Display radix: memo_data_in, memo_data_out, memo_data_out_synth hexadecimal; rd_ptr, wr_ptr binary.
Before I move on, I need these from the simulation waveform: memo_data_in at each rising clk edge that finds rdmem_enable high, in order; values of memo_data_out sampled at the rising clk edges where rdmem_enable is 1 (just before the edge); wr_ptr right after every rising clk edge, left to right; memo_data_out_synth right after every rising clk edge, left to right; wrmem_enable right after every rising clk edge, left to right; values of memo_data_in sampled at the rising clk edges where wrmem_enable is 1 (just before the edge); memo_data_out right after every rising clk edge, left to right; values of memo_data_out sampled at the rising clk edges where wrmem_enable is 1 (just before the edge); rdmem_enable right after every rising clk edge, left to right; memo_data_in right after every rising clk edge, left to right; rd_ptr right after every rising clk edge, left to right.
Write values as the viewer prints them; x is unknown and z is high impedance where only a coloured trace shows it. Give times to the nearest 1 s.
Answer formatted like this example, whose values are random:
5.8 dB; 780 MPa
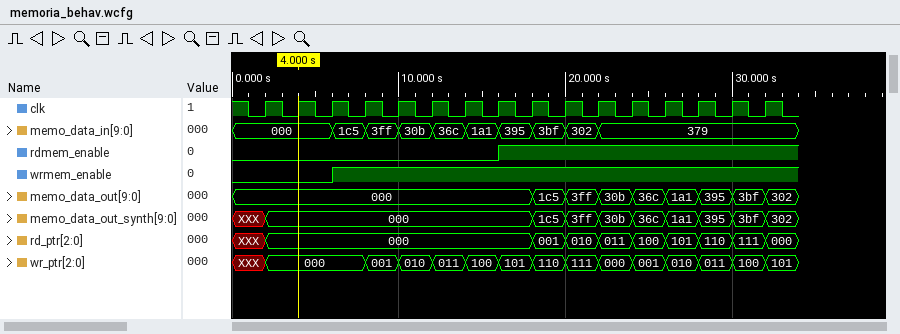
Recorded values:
395, 3bf, 302, 379, 379, 379, 379, 379; 000, 1c5, 3ff, 30b, 36c, 1a1, 395, 3bf; 000, 000, 000, 001, 010, 011, 100, 101, 110, 111, 000, 001, 010, 011, 100, 101; 000, 000, 000, 000, 000, 000, 000, 000, 1c5, 3ff, 30b, 36c, 1a1, 395, 3bf, 302; 0 0 1 1 1 1 1 1 1 1 1 1 1 1 1 1; 1c5, 3ff, 30b, 36c, 1a1, 395, 3bf, 302, 379, 379, 379, 379, 379; 000, 000, 000, 000, 000, 000, 000, 000, 1c5, 3ff, 30b, 36c, 1a1, 395, 3bf, 302; 000, 000, 000, 000, 000, 000, 1c5, 3ff, 30b, 36c, 1a1, 395, 3bf; 0 0 0 0 0 0 0 1 1 1 1 1 1 1 1 1; 000, 000, 1c5, 3ff, 30b, 36c, 1a1, 395, 3bf, 302, 379, 379, 379, 379, 379, 379; 000, 000, 000, 000, 000, 000, 000, 000, 001, 010, 011, 100, 101, 110, 111, 000
